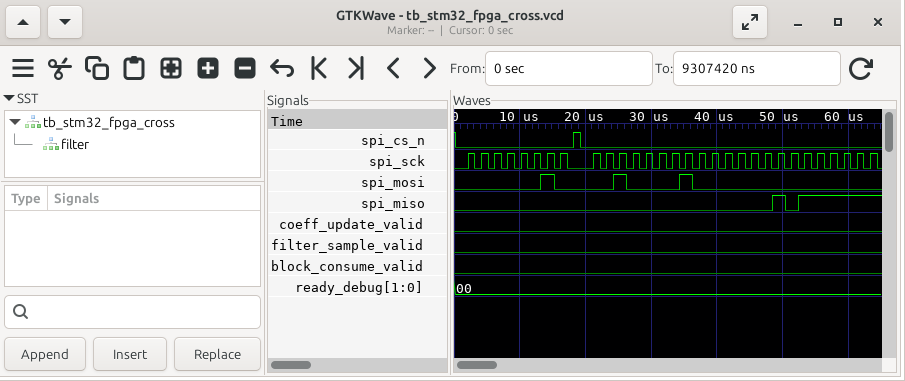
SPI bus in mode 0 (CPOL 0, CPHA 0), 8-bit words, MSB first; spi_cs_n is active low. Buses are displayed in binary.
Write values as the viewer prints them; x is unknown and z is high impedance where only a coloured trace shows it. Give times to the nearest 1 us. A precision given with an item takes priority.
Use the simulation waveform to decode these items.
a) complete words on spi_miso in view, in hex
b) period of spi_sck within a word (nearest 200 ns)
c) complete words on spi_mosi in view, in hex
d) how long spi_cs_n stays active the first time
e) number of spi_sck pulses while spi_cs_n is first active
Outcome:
00, 00, 02
2000 ns
02, 21, 00
18 us
8
